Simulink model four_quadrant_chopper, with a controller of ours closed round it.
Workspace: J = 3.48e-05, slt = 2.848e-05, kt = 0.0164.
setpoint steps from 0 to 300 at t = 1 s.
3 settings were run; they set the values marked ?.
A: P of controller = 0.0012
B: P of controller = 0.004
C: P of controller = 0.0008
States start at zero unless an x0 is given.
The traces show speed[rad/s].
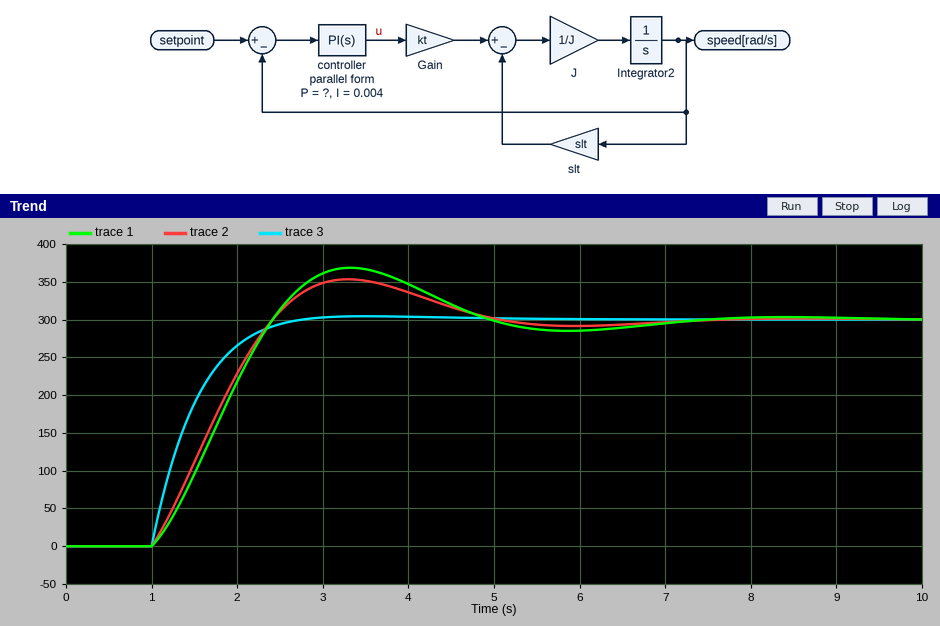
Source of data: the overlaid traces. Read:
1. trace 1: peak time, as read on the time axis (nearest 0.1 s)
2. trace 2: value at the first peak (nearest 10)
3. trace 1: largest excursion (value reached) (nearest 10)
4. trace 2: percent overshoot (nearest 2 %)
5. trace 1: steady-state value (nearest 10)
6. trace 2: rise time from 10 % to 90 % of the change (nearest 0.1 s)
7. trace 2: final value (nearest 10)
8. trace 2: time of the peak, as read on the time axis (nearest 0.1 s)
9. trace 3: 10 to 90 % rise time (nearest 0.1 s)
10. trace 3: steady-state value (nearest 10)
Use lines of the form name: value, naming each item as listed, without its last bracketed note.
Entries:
trace 1: peak time, as read on the time axis: 3.3 s
trace 2: value at the first peak: 350
trace 1: largest excursion (value reached): 370
trace 2: percent overshoot: 18 %
trace 1: steady-state value: 300
trace 2: rise time from 10 % to 90 % of the change: 1.1 s
trace 2: final value: 300
trace 2: time of the peak, as read on the time axis: 3.3 s
trace 3: 10 to 90 % rise time: 1.0 s
trace 3: steady-state value: 300
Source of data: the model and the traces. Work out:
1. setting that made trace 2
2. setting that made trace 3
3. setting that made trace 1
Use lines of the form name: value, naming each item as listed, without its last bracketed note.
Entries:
setting that made trace 2: A
setting that made trace 3: B
setting that made trace 1: C
